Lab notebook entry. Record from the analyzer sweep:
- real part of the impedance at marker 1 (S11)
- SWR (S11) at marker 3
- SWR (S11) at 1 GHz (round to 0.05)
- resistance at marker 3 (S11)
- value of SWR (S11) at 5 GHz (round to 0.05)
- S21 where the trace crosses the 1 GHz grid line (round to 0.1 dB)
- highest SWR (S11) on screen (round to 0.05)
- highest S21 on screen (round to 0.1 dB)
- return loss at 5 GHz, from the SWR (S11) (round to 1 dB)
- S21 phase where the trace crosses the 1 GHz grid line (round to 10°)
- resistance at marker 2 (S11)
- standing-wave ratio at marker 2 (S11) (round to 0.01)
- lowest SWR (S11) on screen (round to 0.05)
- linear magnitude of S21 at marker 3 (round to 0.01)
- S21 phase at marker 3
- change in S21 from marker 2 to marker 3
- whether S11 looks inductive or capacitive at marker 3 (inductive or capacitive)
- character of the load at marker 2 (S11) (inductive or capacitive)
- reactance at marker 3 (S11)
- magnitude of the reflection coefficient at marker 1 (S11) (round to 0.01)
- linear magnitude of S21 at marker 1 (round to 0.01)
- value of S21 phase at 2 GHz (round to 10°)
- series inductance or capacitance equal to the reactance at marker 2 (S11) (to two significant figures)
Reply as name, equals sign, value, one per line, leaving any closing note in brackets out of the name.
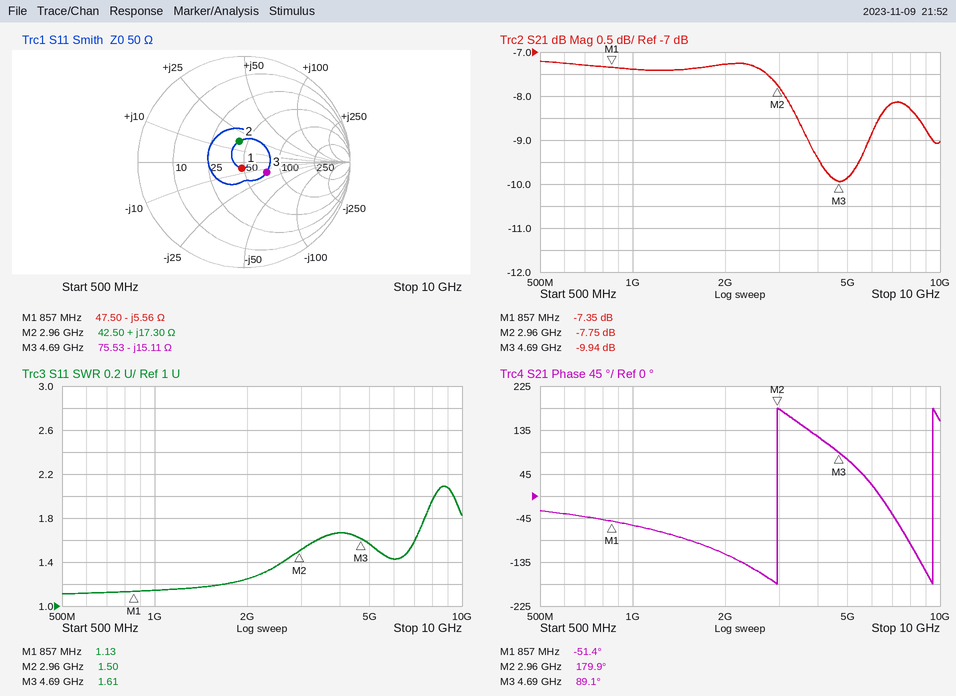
real part of the impedance at marker 1 = 47.50 Ω
SWR (S11) at marker 3 = 1.61
SWR (S11) at 1 GHz = 1.15
resistance at marker 3 = 75.53 Ω
value of SWR (S11) at 5 GHz = 1.55
S21 where the trace crosses the 1 GHz grid line = -7.4 dB
highest SWR (S11) on screen = 2.10
highest S21 on screen = -7.2 dB
return loss at 5 GHz, from the SWR (S11) = 13 dB
S21 phase where the trace crosses the 1 GHz grid line = -60°
resistance at marker 2 = 42.50 Ω
standing-wave ratio at marker 2 (S11) = 1.50
lowest SWR (S11) on screen = 1.10
linear magnitude of S21 at marker 3 = 0.32
S21 phase at marker 3 = 89.1°
change in S21 from marker 2 to marker 3 = -2.19 dB
whether S11 looks inductive or capacitive at marker 3 = capacitive
character of the load at marker 2 (S11) = inductive
reactance at marker 3 = -15.11 Ω
magnitude of the reflection coefficient at marker 1 (S11) = 0.06
linear magnitude of S21 at marker 1 = 0.43
value of S21 phase at 2 GHz = -120°
series inductance or capacitance equal to the reactance at marker 2 (S11) = 930 pH
